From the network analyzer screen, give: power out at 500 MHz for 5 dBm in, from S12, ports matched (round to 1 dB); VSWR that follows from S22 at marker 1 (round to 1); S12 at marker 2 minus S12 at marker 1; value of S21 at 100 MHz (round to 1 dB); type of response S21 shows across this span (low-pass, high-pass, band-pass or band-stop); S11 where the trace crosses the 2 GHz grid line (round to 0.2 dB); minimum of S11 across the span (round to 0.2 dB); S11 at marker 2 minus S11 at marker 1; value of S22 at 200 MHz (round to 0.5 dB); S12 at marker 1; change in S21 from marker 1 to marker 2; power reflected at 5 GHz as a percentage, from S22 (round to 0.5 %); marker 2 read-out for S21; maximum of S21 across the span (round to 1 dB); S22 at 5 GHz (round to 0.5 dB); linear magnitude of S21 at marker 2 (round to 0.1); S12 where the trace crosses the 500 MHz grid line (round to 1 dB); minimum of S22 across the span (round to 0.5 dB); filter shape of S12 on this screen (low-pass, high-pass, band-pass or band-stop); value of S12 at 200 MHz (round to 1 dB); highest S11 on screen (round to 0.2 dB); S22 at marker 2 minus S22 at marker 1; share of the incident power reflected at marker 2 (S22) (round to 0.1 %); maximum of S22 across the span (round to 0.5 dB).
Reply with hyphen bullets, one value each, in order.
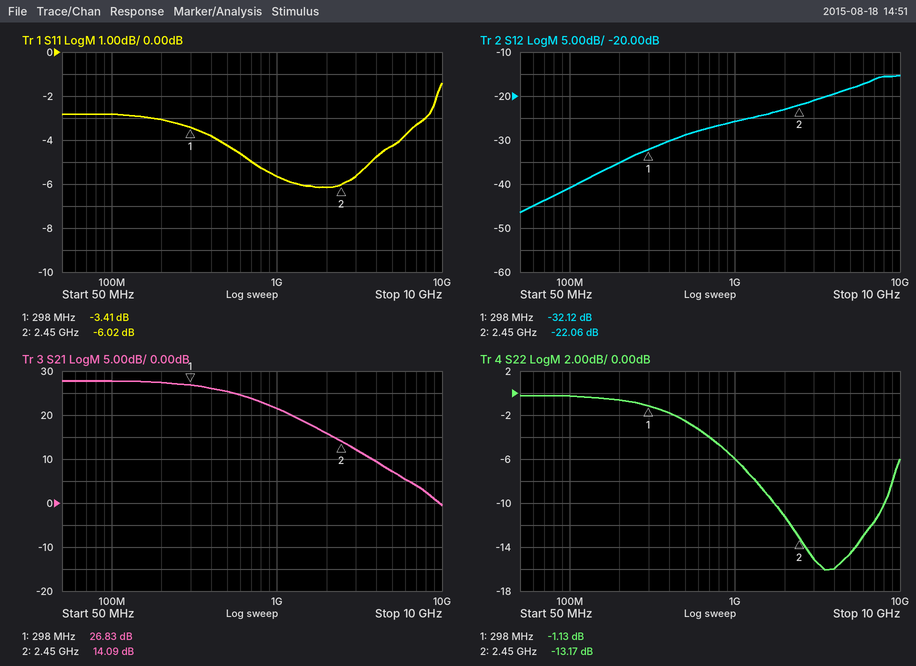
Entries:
- -24 dBm
- 15
- 10.06 dB
- 28 dB
- low-pass
- -6.2 dB
- -6.2 dB
- -2.61 dB
- -0.5 dB
- -32.12 dB
- -12.74 dB
- 3.5 %
- 14.09 dB
- 28 dB
- -14.5 dB
- 5.1
- -29 dB
- -16.0 dB
- high-pass
- -35 dB
- -1.4 dB
- -12.04 dB
- 4.8 %
- 0.0 dB
